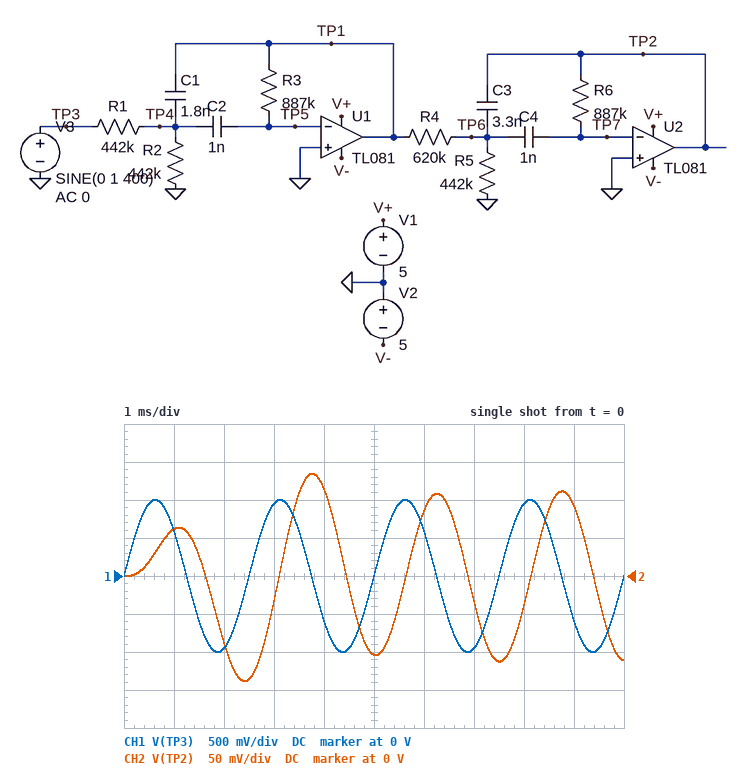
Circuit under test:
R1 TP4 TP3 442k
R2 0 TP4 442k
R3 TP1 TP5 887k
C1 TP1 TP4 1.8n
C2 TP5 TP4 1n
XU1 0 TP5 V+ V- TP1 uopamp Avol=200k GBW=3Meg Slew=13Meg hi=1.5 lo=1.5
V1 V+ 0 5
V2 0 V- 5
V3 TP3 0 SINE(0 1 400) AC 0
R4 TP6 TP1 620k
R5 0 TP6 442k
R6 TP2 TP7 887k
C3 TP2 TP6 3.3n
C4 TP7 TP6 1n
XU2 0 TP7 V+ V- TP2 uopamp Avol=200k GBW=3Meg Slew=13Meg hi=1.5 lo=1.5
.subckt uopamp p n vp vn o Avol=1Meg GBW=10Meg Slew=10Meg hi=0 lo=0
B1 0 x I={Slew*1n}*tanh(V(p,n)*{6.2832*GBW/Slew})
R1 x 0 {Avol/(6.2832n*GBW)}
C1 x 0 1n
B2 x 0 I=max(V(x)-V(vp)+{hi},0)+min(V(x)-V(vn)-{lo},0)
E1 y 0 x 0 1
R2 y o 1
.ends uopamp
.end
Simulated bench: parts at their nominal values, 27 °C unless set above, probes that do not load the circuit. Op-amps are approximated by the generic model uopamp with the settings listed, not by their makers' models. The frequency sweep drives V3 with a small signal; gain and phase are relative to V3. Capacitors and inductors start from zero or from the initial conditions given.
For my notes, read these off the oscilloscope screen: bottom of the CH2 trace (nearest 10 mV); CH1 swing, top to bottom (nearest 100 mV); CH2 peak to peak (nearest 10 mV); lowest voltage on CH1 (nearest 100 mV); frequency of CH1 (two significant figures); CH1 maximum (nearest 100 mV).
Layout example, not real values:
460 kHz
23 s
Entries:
-140 mV
2.0 V
270 mV
-1.0 V
400 Hz
1.0 V
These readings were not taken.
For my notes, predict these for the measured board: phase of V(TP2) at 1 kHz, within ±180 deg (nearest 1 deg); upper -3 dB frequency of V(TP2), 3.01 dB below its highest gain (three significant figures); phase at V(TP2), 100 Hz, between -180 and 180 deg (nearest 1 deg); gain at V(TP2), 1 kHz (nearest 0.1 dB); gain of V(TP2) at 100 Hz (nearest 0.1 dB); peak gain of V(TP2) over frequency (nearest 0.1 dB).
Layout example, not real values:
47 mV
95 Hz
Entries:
-150 deg
338 Hz
111 deg
-35.8 dB
-23.2 dB
-13.3 dB
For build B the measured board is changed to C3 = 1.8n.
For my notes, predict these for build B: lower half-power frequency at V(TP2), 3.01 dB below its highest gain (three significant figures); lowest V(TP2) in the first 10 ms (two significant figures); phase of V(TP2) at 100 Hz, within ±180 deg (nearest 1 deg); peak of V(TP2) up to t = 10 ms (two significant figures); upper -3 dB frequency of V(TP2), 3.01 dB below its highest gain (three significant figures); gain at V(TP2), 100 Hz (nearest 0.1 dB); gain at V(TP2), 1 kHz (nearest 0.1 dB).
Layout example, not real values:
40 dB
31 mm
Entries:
183 Hz
-230 mV
127 deg
260 mV
364 Hz
-22.9 dB
-30.4 dB
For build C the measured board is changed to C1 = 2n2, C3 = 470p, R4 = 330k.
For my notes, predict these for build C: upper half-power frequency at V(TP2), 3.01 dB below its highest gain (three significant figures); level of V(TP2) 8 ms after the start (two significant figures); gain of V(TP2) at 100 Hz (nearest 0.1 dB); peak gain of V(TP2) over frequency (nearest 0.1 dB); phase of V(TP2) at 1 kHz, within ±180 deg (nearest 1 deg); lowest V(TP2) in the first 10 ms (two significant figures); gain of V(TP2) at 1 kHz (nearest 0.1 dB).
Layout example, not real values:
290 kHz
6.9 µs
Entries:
645 Hz
600 mV
-20.4 dB
-3.5 dB
-125 deg
-680 mV
-14.2 dB
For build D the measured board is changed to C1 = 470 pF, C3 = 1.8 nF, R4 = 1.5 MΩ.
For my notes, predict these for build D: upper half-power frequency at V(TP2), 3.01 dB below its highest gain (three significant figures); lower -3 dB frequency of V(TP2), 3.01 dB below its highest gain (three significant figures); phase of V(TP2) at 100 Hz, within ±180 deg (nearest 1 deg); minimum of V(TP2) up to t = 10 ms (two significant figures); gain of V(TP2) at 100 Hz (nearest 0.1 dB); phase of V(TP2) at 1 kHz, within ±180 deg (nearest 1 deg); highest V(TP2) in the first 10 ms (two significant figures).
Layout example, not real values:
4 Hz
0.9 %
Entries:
612 Hz
206 Hz
131 deg
-180 mV
-28.8 dB
-126 deg
190 mV
